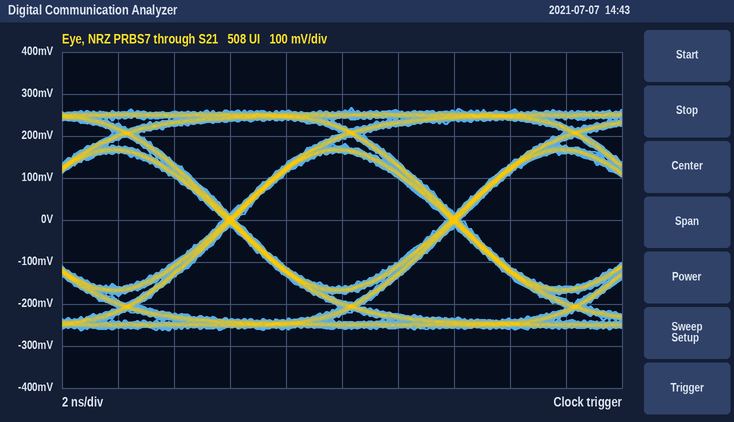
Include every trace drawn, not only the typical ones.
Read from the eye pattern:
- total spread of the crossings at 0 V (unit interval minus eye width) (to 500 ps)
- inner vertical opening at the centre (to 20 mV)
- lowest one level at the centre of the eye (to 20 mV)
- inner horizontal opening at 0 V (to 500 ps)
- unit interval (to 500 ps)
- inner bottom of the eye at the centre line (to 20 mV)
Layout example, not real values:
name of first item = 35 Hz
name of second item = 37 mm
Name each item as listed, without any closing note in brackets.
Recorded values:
total spread of the crossings at 0 V (unit interval minus eye width) = 500 ps
inner vertical opening at the centre = 320 mV
lowest one level at the centre of the eye = 160 mV
inner horizontal opening at 0 V = 7.5 ns
unit interval = 8.0 ns
inner bottom of the eye at the centre line = -160 mV
